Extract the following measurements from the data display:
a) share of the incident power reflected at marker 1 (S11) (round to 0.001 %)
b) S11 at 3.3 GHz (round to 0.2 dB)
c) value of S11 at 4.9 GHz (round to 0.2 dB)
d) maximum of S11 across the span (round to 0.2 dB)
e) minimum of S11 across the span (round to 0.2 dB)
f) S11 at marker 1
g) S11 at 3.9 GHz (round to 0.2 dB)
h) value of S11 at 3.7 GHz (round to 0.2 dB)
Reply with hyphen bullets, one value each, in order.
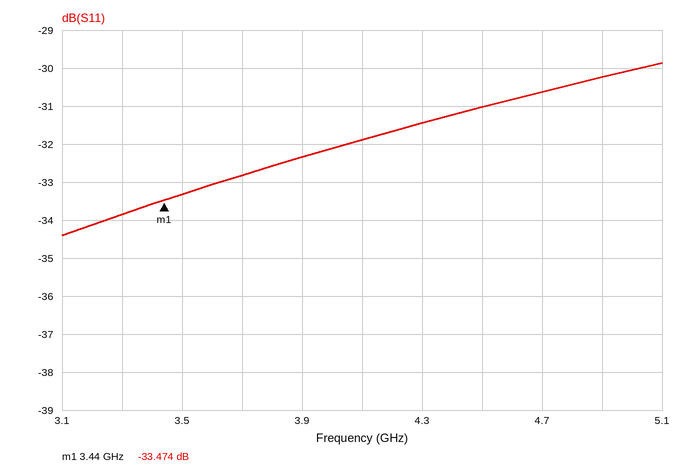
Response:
- 0.045 %
- -33.8 dB
- -30.2 dB
- -29.8 dB
- -34.4 dB
- -33.474 dB
- -32.4 dB
- -32.8 dB
